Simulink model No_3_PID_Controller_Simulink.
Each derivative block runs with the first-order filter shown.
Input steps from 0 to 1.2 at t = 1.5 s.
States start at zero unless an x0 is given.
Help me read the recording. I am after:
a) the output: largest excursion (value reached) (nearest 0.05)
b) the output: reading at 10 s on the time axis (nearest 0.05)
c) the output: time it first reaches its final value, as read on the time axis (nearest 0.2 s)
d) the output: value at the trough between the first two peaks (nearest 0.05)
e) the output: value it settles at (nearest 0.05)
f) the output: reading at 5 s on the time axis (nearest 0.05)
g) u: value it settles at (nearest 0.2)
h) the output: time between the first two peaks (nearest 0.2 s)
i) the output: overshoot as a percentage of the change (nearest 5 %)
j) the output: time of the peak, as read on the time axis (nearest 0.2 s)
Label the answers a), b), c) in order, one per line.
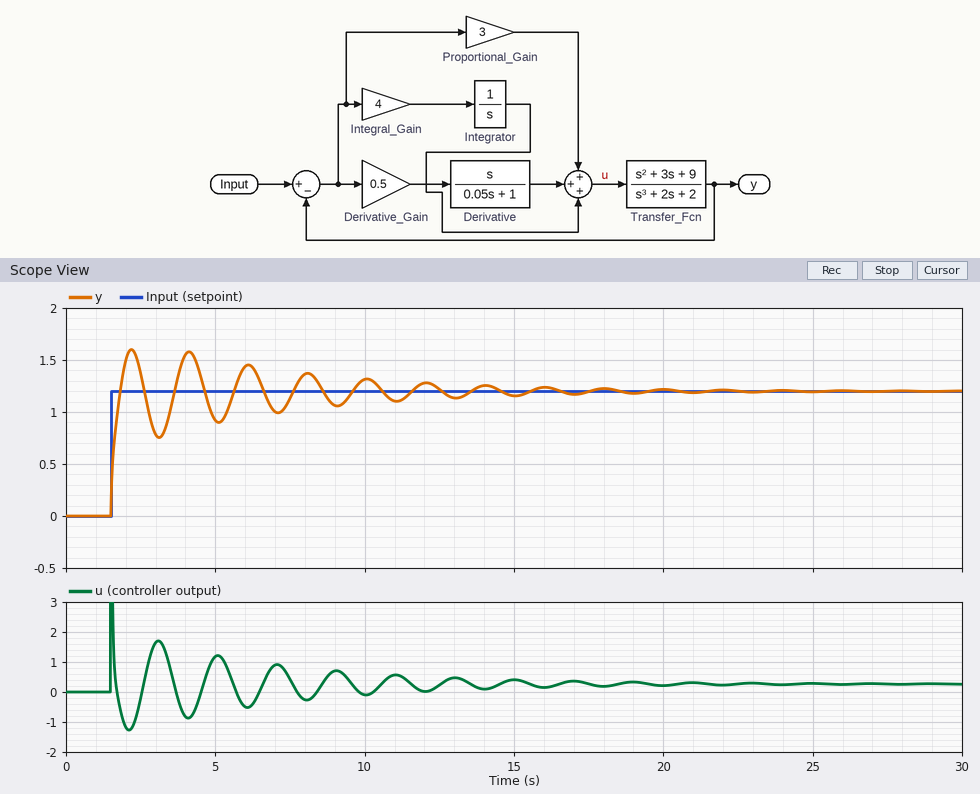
a) 1.60
b) 1.30
c) 1.8 s
d) 0.75
e) 1.20
f) 0.90
g) 0.2
h) 2.0 s
i) 35 %
j) 2.2 s
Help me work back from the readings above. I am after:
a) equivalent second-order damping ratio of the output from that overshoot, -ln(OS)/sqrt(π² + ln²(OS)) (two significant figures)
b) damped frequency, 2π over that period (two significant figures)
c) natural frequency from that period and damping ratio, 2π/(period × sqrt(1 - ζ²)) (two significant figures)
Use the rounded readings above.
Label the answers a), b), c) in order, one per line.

a) 0.32
b) 3.1 rad/s
c) 3.3 rad/s
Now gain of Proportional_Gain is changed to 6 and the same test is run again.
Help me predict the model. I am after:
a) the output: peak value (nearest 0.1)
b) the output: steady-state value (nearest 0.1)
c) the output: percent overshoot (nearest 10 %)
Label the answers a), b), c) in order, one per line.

a) 1.5
b) 1.2
c) 20 %
